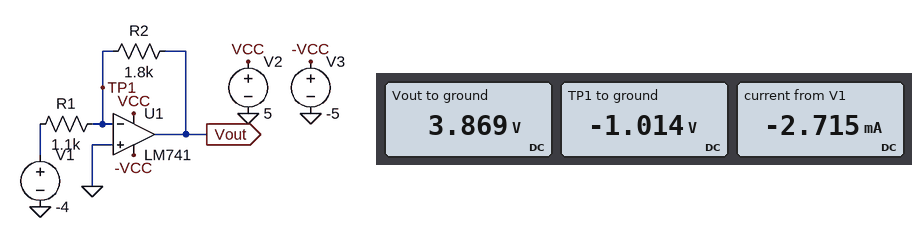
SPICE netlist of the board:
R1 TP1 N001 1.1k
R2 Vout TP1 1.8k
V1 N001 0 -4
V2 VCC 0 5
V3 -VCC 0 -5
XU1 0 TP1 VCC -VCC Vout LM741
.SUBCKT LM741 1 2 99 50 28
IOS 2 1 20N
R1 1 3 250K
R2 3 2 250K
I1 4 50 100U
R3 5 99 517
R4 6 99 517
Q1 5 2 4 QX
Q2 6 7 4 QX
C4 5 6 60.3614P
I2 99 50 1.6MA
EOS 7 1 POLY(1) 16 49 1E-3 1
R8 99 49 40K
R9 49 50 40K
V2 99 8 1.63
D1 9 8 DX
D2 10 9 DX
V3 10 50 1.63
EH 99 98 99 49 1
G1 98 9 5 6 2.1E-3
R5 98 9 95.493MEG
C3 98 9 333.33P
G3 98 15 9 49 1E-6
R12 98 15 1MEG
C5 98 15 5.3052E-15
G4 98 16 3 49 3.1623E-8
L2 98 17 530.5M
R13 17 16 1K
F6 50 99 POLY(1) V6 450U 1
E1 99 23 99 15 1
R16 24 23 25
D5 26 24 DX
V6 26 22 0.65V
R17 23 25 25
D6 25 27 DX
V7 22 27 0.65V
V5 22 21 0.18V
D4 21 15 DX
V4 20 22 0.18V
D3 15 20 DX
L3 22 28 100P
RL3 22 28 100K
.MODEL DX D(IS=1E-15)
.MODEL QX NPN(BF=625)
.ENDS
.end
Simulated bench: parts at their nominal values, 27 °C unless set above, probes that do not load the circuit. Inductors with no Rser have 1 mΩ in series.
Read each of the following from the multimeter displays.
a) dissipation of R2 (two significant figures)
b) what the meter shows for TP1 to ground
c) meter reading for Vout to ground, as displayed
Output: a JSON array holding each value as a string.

["13 mW", "-1.014 V", "3.869 V"]
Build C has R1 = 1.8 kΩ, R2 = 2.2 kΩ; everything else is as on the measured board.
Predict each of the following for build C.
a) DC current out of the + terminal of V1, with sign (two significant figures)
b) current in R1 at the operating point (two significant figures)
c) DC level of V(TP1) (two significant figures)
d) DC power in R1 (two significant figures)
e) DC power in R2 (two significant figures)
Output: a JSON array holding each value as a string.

["-2.0 mA", "2.0 mA", "-450 mV", "7.0 mW", "8.6 mW"]
